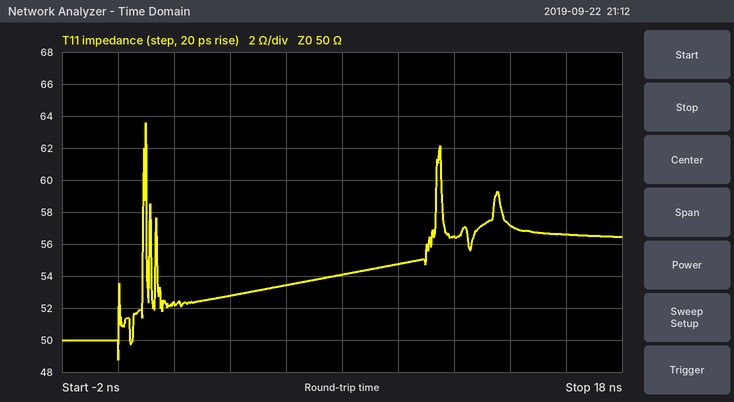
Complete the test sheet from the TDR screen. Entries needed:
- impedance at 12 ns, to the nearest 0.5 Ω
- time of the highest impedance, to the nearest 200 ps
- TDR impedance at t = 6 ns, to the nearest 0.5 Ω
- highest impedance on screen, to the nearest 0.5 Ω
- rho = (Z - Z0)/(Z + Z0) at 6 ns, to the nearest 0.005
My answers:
56.5 Ω
1.0 ns
53.5 Ω
63.5 Ω
+0.035
